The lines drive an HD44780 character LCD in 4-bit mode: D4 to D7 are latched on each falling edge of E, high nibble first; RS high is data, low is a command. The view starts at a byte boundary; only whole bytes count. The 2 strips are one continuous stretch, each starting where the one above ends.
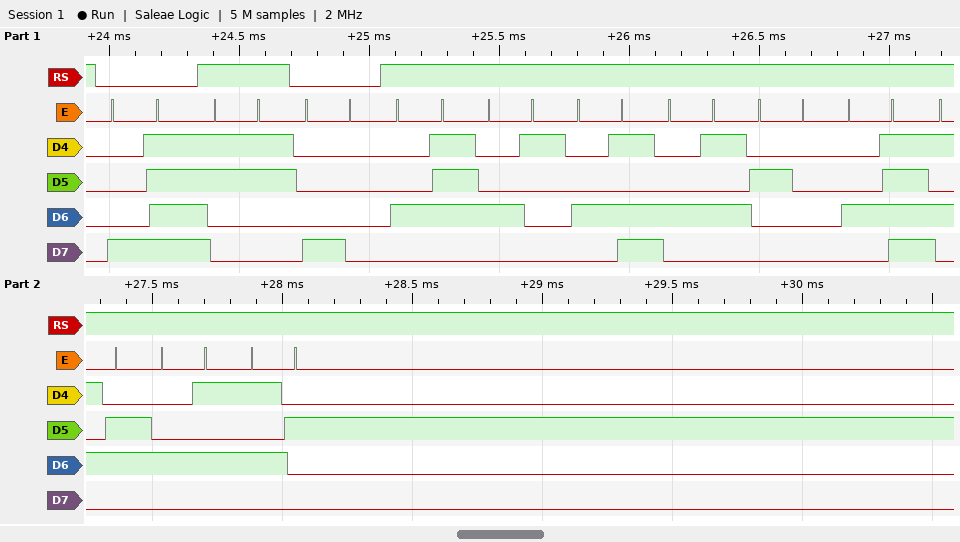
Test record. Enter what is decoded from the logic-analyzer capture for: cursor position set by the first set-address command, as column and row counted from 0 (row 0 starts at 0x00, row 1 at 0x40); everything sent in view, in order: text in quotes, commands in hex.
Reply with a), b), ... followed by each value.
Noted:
a) column 15, row 0
b) 0x8F "3" 0x80 "GAME OVER"
